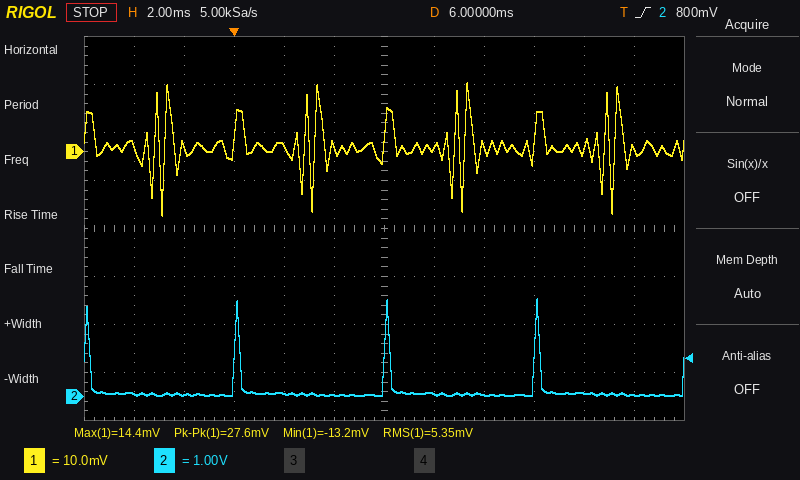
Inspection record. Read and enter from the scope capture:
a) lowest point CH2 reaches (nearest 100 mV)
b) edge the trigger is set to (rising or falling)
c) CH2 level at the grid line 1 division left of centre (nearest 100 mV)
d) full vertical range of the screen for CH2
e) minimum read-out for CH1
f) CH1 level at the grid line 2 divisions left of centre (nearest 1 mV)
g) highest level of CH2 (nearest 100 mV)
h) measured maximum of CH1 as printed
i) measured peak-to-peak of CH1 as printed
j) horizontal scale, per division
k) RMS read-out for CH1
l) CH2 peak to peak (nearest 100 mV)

0.0 V
rising
0.0 V
8 V
-13.2 mV
1 mV
2.0 V
14.4 mV
27.6 mV
2 ms
5.35 mV
2.0 V
